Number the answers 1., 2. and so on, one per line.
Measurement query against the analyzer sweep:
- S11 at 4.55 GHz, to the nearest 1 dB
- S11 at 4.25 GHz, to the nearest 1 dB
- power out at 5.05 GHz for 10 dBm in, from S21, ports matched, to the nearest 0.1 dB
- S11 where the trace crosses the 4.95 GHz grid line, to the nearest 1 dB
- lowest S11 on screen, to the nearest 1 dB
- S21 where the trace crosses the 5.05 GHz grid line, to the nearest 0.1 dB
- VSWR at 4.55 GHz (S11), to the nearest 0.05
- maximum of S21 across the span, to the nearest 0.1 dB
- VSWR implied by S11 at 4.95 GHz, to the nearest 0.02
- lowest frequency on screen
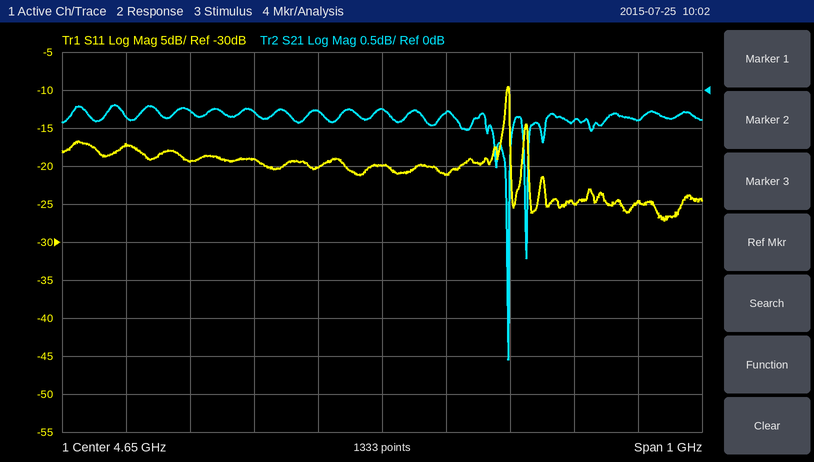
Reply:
1. -20 dB
2. -17 dB
3. 9.6 dBm
4. -25 dB
5. -27 dB
6. -0.4 dB
7. 1.20
8. -0.2 dB
9. 1.12
10. 4.15 GHz
